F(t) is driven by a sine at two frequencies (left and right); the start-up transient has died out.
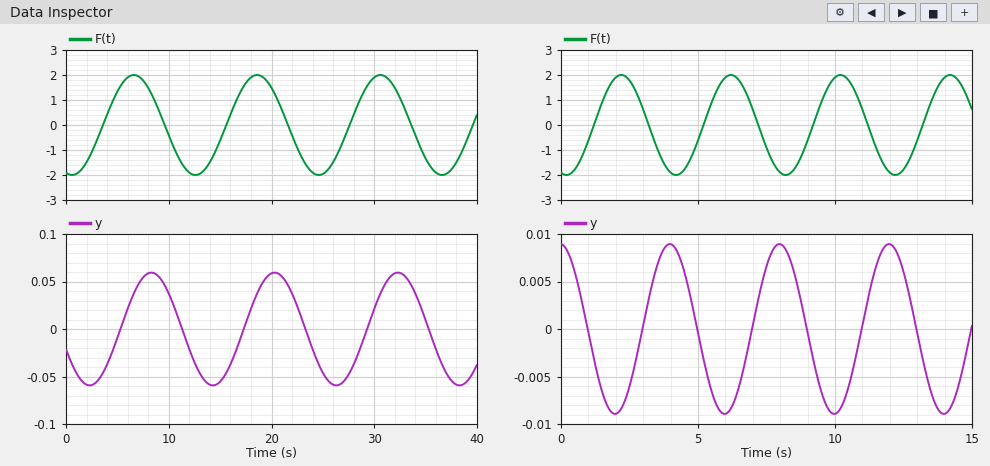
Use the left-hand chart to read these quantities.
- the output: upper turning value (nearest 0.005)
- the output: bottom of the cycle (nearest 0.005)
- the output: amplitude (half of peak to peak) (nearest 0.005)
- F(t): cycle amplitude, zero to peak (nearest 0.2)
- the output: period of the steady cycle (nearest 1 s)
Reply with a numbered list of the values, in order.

1. 0.060
2. -0.060
3. 0.060
4. 2.0
5. 12 s
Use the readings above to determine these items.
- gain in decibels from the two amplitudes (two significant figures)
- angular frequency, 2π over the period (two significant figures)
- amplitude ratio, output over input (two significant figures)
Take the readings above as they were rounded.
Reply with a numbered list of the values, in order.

1. -30 dB
2. 0.52 rad/s
3. 0.030
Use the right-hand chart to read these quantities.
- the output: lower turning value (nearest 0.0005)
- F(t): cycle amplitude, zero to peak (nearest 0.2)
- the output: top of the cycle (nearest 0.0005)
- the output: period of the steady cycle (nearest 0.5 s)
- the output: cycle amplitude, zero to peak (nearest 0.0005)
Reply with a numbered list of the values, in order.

1. -0.0090
2. 2.0
3. 0.0090
4. 4.0 s
5. 0.0090
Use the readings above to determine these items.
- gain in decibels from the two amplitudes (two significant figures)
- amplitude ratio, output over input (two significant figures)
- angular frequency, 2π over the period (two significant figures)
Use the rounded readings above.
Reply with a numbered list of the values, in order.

1. -47 dB
2. 0.0045
3. 1.6 rad/s
